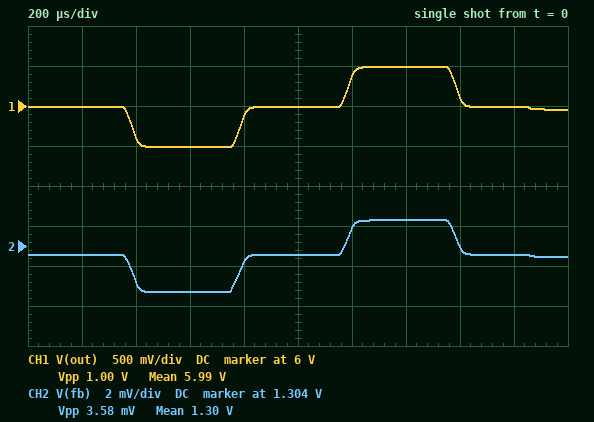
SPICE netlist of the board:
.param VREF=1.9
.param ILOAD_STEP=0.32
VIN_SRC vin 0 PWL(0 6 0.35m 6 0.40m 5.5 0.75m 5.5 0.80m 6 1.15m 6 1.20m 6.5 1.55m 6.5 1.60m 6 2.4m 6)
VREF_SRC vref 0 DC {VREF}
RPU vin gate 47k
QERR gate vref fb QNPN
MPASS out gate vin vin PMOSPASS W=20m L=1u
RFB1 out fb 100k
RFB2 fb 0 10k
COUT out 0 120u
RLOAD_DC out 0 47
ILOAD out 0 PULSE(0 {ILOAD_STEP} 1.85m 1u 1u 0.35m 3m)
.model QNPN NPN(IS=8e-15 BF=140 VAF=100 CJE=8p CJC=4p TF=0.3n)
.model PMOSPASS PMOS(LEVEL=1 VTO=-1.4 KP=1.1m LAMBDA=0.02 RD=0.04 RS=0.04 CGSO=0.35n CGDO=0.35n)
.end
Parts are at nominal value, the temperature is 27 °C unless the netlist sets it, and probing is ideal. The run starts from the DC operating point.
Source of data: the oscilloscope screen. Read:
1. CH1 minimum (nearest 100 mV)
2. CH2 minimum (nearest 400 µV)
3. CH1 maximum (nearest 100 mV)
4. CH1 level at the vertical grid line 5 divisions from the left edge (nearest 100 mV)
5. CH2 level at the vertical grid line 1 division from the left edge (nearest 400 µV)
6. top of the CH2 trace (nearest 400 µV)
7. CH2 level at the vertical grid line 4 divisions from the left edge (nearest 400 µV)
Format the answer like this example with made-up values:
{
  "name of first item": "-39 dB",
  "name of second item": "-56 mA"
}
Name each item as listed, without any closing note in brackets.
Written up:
{
  "CH1 minimum": "5.5 V",
  "CH2 minimum": "1.3016 V",
  "CH1 maximum": "6.5 V",
  "CH1 level at the vertical grid line 5 divisions from the left edge": "6.0 V",
  "CH2 level at the vertical grid line 1 division from the left edge": "1.3036 V",
  "top of the CH2 trace": "1.3052 V",
  "CH2 level at the vertical grid line 4 divisions from the left edge": "1.3032 V"
}
